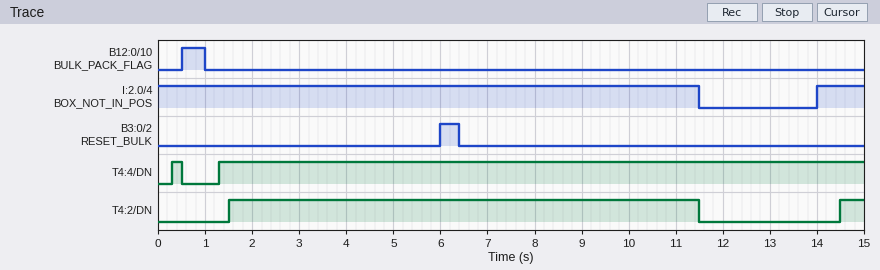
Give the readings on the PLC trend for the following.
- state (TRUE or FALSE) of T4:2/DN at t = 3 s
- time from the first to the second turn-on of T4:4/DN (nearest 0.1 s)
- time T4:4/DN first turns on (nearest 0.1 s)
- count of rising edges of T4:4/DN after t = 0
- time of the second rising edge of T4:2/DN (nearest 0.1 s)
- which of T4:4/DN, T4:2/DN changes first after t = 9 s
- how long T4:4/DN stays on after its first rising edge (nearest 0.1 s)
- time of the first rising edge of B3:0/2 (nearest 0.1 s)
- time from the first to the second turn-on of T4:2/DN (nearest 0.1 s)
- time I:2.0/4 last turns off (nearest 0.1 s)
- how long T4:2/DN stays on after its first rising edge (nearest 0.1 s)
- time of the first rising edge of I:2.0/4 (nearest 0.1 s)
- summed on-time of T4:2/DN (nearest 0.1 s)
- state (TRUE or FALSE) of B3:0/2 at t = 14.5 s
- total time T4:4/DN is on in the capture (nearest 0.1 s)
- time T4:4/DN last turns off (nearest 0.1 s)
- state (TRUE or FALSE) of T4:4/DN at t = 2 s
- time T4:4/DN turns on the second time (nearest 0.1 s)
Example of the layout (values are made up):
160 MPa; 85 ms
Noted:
TRUE; 1.0 s; 0.3 s; 2; 14.5 s; T4:2/DN; 0.2 s; 6.0 s; 13.0 s; 11.5 s; 10.0 s; 14.0 s; 10.5 s; FALSE; 13.9 s; 0.5 s; TRUE; 1.3 s
